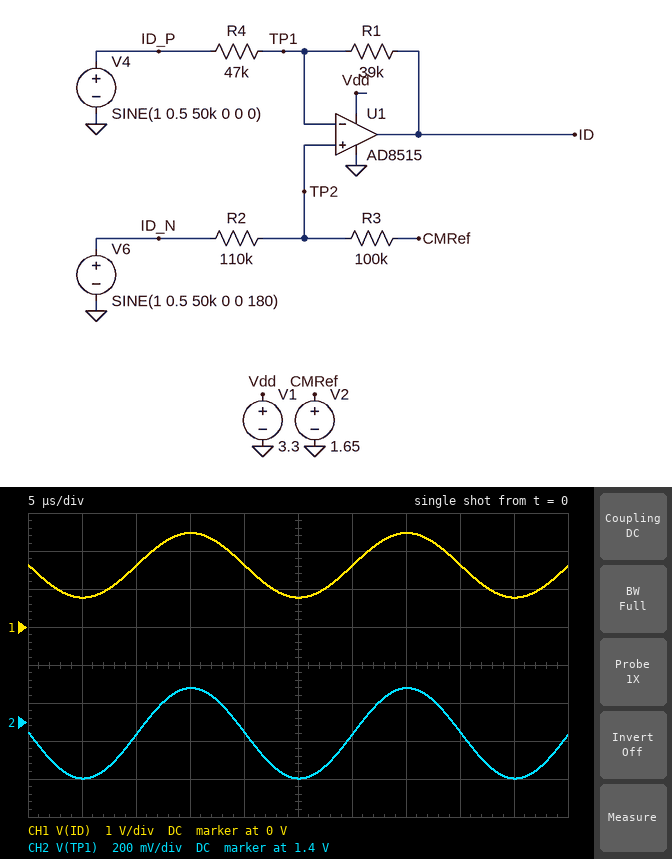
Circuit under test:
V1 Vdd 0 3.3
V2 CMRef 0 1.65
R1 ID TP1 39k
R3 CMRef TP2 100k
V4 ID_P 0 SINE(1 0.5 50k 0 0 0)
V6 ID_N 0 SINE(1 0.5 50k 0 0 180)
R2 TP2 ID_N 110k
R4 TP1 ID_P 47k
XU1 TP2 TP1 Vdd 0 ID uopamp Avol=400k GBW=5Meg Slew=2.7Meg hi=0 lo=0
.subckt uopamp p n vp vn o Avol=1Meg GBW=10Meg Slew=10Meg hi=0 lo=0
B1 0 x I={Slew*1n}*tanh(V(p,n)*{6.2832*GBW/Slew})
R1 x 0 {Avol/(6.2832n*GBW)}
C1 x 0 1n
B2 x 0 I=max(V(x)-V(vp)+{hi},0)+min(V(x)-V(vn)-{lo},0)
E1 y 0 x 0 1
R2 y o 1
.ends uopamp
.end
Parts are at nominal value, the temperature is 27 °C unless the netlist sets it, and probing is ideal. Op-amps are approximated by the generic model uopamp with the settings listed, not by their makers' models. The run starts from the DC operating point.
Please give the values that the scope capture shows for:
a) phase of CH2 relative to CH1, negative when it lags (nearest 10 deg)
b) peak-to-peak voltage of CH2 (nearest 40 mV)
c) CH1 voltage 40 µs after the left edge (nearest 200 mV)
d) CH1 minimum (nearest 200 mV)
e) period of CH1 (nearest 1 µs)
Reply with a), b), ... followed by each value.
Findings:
a) 0 deg
b) 480 mV
c) 1.6 V
d) 800 mV
e) 20 µs
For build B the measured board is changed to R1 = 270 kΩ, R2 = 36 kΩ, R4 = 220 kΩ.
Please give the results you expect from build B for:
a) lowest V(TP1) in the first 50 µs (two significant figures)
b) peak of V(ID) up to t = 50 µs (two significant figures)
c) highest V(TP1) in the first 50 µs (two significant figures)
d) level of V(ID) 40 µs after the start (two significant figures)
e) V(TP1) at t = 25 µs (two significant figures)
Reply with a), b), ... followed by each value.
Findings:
a) 820 mV
b) 2.8 V
c) 1.5 V
d) 1.4 V
e) 830 mV
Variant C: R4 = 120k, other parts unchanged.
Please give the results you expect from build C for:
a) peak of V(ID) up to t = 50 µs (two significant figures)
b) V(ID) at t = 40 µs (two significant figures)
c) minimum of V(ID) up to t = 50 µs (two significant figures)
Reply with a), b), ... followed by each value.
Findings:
a) 1.9 V
b) 1.5 V
c) 970 mV
